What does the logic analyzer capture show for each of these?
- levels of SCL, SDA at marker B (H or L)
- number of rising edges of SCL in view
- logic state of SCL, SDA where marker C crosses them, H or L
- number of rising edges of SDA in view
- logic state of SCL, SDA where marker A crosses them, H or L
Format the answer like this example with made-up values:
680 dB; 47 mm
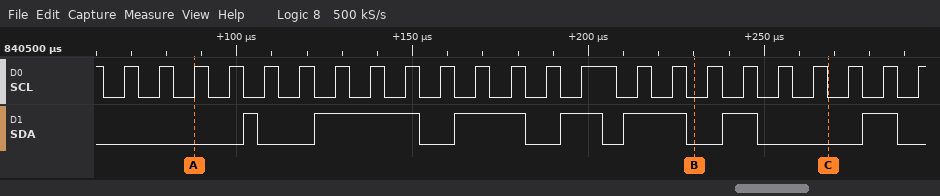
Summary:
SCL=L, SDA=L; 23; SCL=L, SDA=L; 7; SCL=H, SDA=L
